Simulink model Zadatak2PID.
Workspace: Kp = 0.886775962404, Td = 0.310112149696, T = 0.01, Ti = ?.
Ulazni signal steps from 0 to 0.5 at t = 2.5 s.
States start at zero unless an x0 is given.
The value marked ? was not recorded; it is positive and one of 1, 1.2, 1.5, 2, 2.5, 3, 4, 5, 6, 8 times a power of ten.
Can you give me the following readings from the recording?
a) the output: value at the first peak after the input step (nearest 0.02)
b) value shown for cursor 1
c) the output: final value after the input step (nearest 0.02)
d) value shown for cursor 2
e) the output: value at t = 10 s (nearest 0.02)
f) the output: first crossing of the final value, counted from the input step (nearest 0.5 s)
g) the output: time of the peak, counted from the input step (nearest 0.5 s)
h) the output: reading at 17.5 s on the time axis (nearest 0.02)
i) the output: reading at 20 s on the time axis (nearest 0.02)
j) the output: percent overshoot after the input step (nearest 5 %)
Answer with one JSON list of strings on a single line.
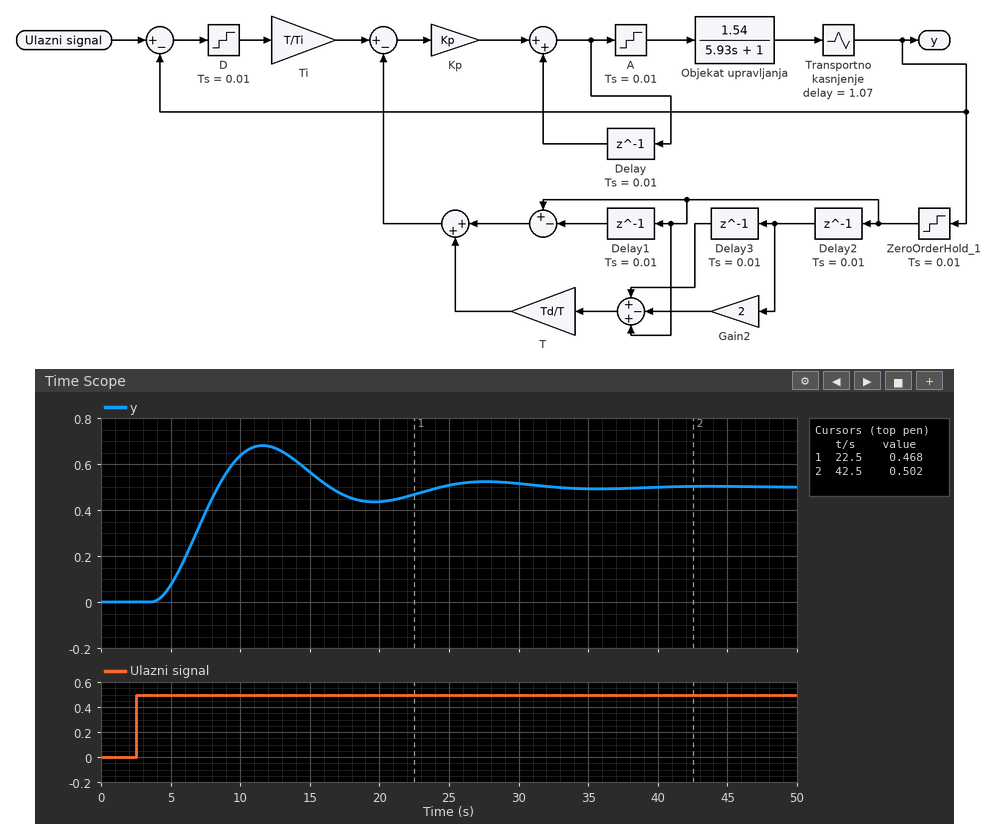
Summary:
["0.68", "0.468", "0.50", "0.502", "0.64", "6.0 s", "9.0 s", "0.46", "0.44", "35 %"]
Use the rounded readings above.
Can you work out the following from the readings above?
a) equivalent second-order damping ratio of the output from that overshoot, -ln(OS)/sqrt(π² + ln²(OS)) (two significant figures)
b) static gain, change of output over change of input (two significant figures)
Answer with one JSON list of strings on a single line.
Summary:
["0.32", "1.0"]
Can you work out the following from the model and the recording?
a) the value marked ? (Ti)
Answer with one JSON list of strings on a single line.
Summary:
["1.5"]
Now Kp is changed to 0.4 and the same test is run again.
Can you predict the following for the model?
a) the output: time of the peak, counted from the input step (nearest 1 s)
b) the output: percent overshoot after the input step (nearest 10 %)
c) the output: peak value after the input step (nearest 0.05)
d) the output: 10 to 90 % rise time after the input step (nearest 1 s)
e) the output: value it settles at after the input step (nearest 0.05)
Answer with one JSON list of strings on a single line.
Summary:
["14 s", "30 %", "0.65", "5 s", "0.50"]
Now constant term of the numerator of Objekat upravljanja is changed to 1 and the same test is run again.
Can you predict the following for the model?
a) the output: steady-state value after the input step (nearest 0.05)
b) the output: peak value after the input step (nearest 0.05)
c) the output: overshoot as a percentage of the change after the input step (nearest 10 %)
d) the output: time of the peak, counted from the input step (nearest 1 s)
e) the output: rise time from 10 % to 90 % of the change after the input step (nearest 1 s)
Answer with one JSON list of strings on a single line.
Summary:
["0.50", "0.65", "30 %", "11 s", "4 s"]
